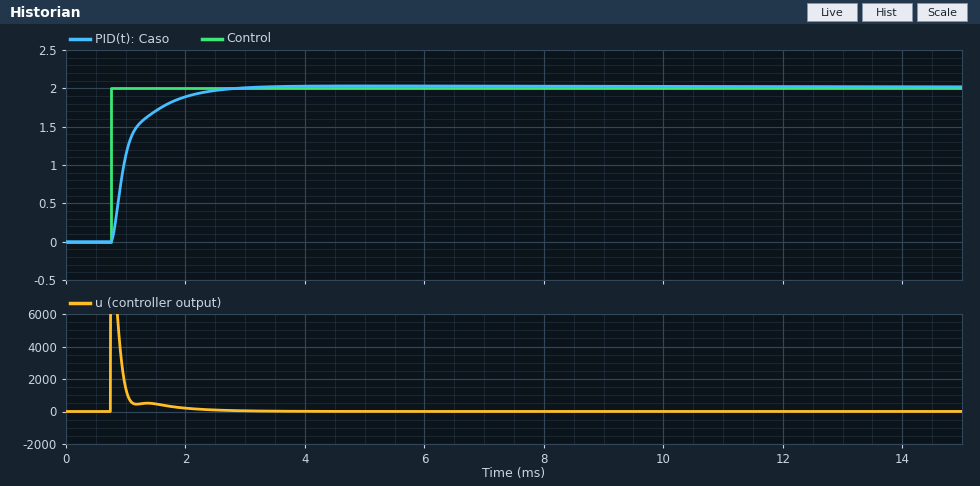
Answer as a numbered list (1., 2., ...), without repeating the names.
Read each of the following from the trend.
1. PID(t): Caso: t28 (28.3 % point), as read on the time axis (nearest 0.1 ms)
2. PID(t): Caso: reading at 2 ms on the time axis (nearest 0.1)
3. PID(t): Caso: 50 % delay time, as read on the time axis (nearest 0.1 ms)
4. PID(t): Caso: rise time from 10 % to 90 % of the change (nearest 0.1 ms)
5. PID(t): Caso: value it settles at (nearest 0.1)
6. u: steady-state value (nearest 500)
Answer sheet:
1. 0.9 ms
2. 1.9
3. 1.0 ms
4. 0.9 ms
5. 2.0
6. 0
